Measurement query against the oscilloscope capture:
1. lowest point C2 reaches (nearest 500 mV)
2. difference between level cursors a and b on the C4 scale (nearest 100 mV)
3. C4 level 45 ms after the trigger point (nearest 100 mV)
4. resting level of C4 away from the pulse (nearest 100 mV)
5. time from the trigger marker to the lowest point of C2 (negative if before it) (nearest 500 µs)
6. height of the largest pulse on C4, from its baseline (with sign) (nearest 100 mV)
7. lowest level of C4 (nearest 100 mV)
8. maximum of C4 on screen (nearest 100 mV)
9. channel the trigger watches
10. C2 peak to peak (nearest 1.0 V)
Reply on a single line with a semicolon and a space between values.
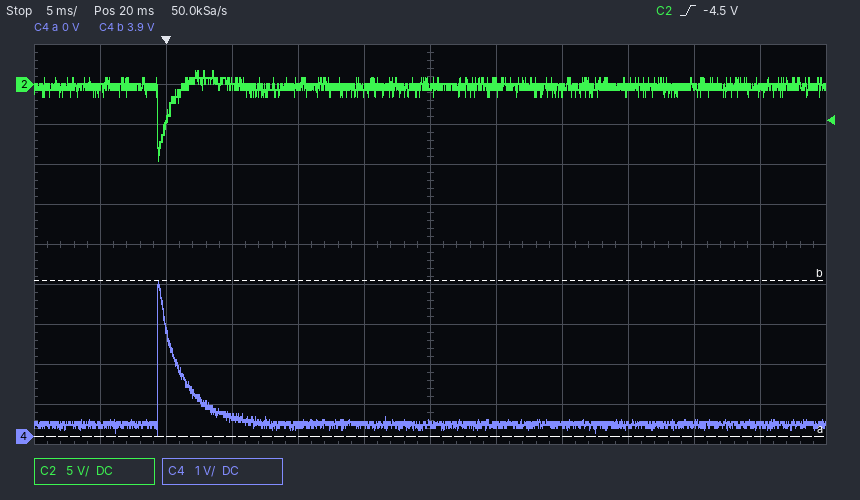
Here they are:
-9.5 V; 3.9 V; 300 mV; 300 mV; -500 µs; +3.6 V; 0.0 V; 3.9 V; C2; 11.0 V
